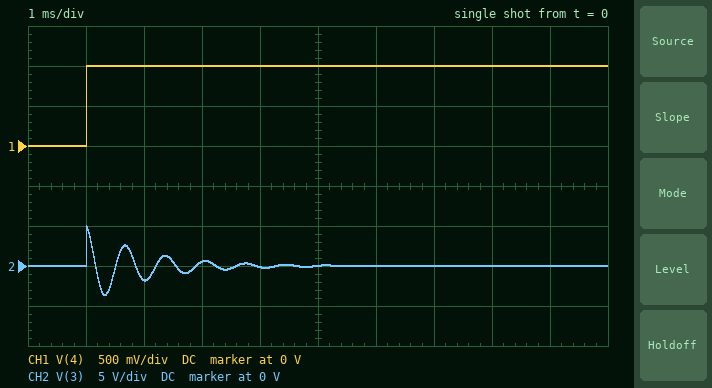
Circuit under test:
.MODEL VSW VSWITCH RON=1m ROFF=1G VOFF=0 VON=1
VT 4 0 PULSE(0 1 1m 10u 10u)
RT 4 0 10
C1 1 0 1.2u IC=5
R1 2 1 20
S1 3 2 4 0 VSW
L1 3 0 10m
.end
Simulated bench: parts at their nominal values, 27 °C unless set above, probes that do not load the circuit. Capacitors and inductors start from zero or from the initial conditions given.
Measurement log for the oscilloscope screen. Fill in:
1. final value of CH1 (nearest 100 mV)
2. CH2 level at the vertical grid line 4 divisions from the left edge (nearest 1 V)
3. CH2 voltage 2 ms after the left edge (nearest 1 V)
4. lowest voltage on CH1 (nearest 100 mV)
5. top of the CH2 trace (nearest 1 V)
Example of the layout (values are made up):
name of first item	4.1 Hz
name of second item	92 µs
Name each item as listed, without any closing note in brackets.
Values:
final value of CH1	1.0 V
CH2 level at the vertical grid line 4 divisions from the left edge	0 V
CH2 voltage 2 ms after the left edge	-2 V
lowest voltage on CH1	0 V
top of the CH2 trace	5 V
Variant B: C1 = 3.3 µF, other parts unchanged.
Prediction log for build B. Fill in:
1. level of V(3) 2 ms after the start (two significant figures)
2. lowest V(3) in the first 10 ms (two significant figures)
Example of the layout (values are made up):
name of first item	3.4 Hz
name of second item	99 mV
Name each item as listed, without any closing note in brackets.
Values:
level of V(3) 2 ms after the start	1.4 V
lowest V(3) in the first 10 ms	-3.0 V
